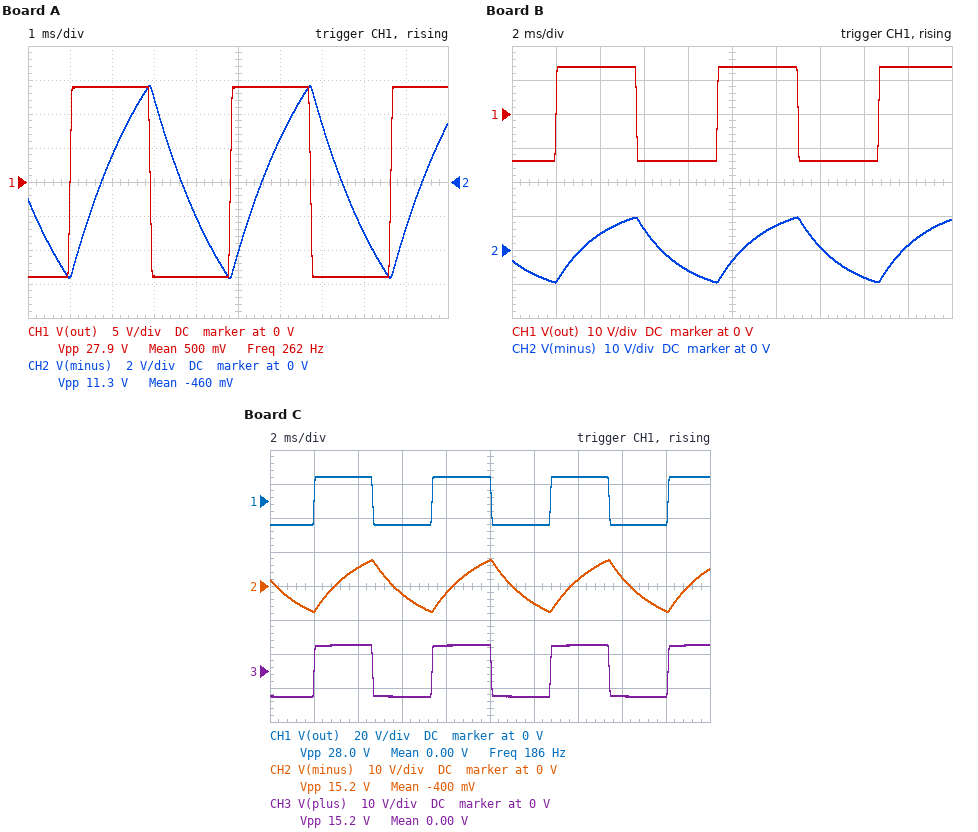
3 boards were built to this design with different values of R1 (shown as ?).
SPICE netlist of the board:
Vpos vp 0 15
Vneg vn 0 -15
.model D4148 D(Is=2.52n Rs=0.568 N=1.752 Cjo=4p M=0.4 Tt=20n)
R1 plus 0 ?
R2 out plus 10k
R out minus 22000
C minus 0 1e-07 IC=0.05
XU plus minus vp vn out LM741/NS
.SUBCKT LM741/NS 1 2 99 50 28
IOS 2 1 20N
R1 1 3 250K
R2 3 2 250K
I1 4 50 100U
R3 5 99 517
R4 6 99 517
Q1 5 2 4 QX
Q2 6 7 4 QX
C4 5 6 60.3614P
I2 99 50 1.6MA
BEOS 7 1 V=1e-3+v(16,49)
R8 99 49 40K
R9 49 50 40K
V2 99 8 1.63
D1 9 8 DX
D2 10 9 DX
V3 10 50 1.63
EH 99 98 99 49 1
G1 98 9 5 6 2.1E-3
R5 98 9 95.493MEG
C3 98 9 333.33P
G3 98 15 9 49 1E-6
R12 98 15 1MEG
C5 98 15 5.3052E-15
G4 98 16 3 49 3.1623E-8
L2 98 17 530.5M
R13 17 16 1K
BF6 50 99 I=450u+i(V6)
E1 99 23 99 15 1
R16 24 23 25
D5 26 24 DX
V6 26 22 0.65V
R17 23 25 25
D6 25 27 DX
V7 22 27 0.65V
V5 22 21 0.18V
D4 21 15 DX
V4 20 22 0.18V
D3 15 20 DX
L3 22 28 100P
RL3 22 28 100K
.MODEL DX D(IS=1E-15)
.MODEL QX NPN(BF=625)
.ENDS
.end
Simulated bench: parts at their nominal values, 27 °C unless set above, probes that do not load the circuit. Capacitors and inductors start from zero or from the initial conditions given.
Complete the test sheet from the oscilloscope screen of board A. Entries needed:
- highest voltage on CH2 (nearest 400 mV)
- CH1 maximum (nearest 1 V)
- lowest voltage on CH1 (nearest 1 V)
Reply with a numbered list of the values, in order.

1. 5.6 V
2. 14 V
3. -14 V
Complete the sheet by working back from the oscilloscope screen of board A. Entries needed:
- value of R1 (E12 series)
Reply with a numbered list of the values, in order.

1. 6.8 kΩ
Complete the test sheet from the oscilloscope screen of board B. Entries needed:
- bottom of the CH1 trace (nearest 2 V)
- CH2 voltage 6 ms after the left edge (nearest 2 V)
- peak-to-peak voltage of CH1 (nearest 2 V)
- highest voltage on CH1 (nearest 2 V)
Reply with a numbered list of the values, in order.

1. -14 V
2. 6 V
3. 28 V
4. 14 V
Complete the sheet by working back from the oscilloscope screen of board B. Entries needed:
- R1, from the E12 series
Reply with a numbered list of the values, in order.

1. 22 kΩ
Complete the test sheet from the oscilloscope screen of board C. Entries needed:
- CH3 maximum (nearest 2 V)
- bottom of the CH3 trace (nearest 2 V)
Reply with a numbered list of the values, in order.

1. 8 V
2. -8 V
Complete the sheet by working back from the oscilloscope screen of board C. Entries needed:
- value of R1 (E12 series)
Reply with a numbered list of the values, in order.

1. 12 kΩ
